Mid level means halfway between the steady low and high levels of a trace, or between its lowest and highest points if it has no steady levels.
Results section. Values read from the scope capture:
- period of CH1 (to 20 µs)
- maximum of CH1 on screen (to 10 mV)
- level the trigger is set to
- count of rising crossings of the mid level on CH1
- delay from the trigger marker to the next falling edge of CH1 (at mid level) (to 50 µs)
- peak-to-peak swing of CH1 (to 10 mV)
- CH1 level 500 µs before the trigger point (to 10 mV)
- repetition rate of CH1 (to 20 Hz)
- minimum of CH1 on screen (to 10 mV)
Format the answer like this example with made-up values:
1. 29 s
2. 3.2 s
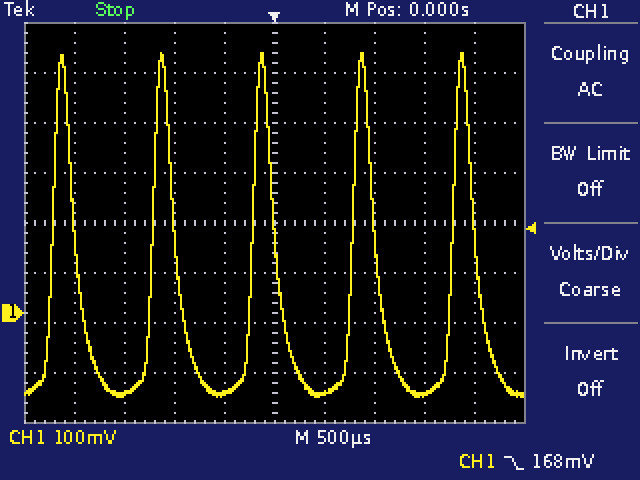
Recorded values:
1. 1.00 ms
2. 520 mV
3. 168 mV
4. 5
5. 1.00 ms
6. 690 mV
7. -160 mV
8. 1.00 kHz
9. -170 mV
